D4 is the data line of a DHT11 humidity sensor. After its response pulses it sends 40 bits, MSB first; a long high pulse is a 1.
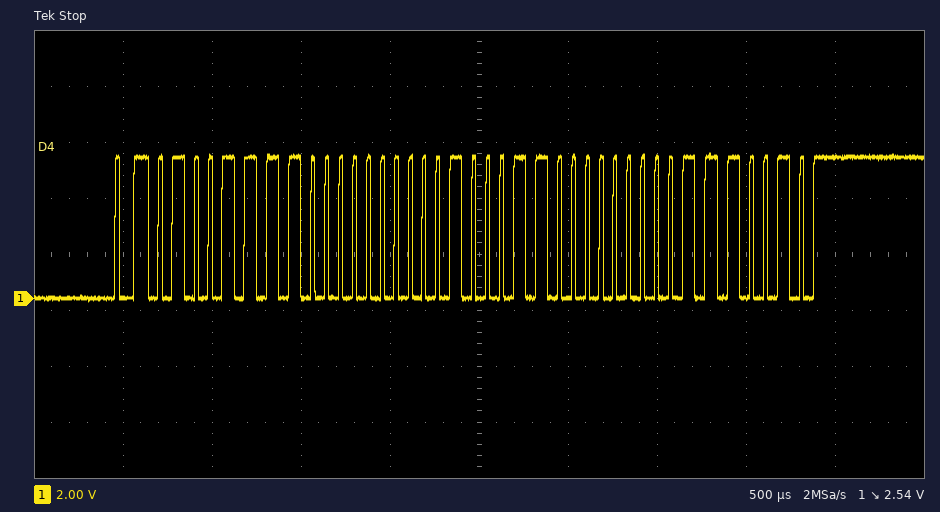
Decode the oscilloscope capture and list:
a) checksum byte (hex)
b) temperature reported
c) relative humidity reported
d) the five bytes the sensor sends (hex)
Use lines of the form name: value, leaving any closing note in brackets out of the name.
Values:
checksum byte: 0x72
temperature reported: 35.0 °C
relative humidity reported: 79 %
the five bytes the sensor sends: 4F 00 23 00 72
